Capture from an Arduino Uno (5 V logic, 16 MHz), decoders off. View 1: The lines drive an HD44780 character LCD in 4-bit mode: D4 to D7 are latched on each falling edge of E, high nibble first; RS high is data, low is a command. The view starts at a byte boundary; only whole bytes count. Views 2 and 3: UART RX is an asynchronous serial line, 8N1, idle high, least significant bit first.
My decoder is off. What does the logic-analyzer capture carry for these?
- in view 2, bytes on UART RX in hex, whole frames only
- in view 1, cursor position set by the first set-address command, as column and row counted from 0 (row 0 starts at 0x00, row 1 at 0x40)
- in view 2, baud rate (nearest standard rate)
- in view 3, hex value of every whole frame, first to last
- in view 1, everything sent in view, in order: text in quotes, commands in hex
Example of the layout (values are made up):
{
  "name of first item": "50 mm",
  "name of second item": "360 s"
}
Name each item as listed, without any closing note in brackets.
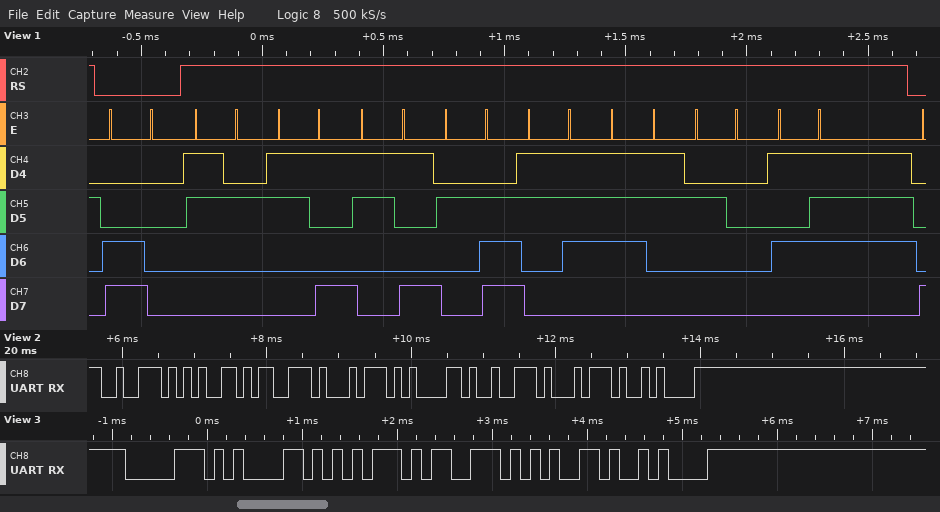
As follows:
{
  "in view 2, bytes on UART RX in hex, whole frames only": "72 65 73 74 61 72 74 0A",
  "in view 1, cursor position set by the first set-address command, as column and row counted from 0": "column 0, row 1",
  "in view 2, baud rate": "9600 baud",
  "in view 3, hex value of every whole frame, first to last": "0x70 0x61 0x75 0x73 0x65 0x0A",
  "in view 1, everything sent in view, in order: text in quotes, commands in hex": "0xC0 \"299.7s W\""
}
